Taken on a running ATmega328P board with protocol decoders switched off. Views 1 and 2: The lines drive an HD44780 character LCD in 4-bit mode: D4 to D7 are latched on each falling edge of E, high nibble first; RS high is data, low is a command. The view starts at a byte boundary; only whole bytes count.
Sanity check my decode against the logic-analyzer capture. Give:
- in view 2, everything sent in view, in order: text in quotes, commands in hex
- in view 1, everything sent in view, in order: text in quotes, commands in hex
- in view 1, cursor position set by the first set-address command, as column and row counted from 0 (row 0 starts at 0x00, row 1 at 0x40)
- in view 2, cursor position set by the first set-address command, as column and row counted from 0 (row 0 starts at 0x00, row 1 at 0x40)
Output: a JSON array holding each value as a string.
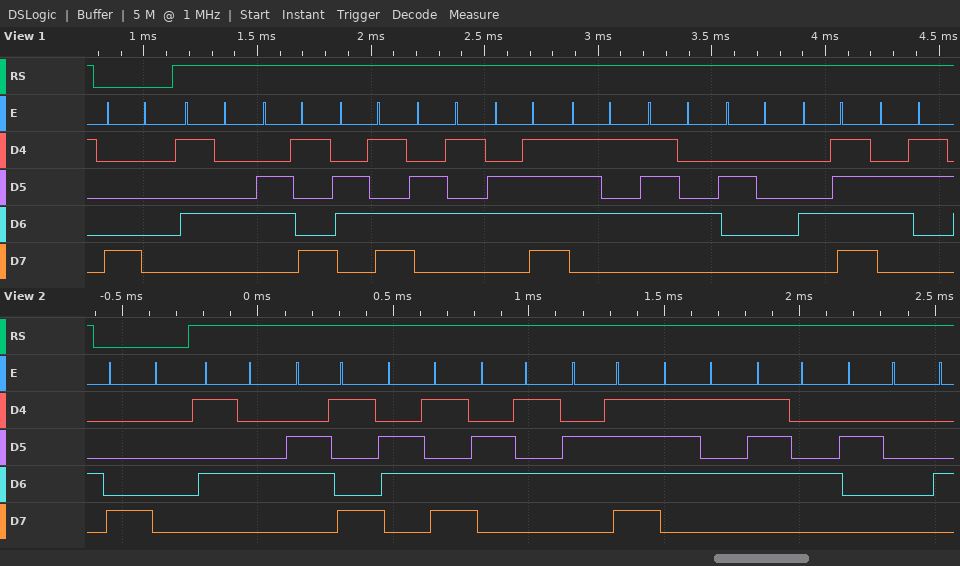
["0x80 \"Timeout \"", "0x80 \"Timeout Oc\"", "column 0, row 0", "column 0, row 0"]
